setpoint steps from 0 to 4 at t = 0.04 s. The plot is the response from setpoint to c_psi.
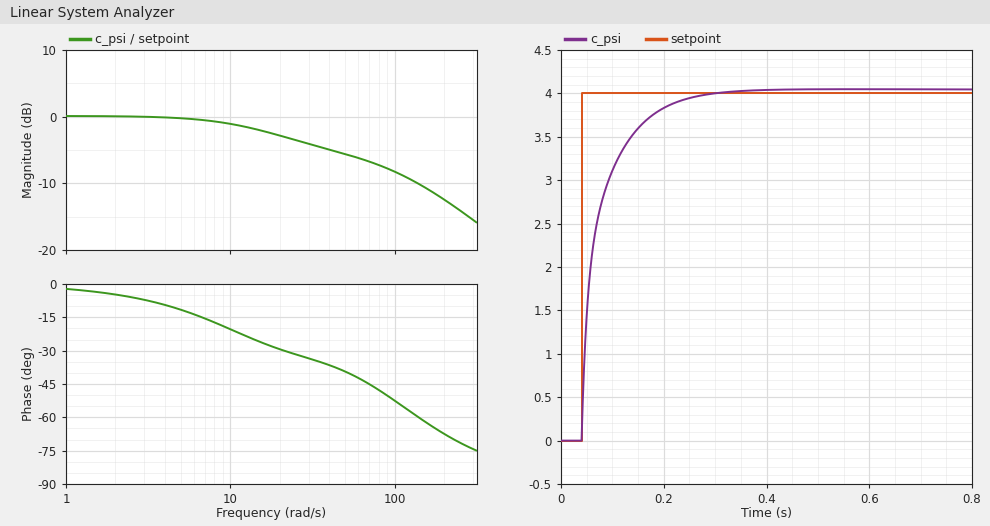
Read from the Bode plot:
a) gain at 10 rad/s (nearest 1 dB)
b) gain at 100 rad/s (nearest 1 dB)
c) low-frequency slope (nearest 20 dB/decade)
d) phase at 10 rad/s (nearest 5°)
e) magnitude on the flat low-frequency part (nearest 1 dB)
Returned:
-1 dB
-8 dB
0 dB/decade
-20°
0 dB
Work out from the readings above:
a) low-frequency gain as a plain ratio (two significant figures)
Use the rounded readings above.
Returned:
1.0
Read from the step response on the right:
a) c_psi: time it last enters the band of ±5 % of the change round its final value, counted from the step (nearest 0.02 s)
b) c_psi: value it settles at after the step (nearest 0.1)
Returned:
0.16 s
4.0
